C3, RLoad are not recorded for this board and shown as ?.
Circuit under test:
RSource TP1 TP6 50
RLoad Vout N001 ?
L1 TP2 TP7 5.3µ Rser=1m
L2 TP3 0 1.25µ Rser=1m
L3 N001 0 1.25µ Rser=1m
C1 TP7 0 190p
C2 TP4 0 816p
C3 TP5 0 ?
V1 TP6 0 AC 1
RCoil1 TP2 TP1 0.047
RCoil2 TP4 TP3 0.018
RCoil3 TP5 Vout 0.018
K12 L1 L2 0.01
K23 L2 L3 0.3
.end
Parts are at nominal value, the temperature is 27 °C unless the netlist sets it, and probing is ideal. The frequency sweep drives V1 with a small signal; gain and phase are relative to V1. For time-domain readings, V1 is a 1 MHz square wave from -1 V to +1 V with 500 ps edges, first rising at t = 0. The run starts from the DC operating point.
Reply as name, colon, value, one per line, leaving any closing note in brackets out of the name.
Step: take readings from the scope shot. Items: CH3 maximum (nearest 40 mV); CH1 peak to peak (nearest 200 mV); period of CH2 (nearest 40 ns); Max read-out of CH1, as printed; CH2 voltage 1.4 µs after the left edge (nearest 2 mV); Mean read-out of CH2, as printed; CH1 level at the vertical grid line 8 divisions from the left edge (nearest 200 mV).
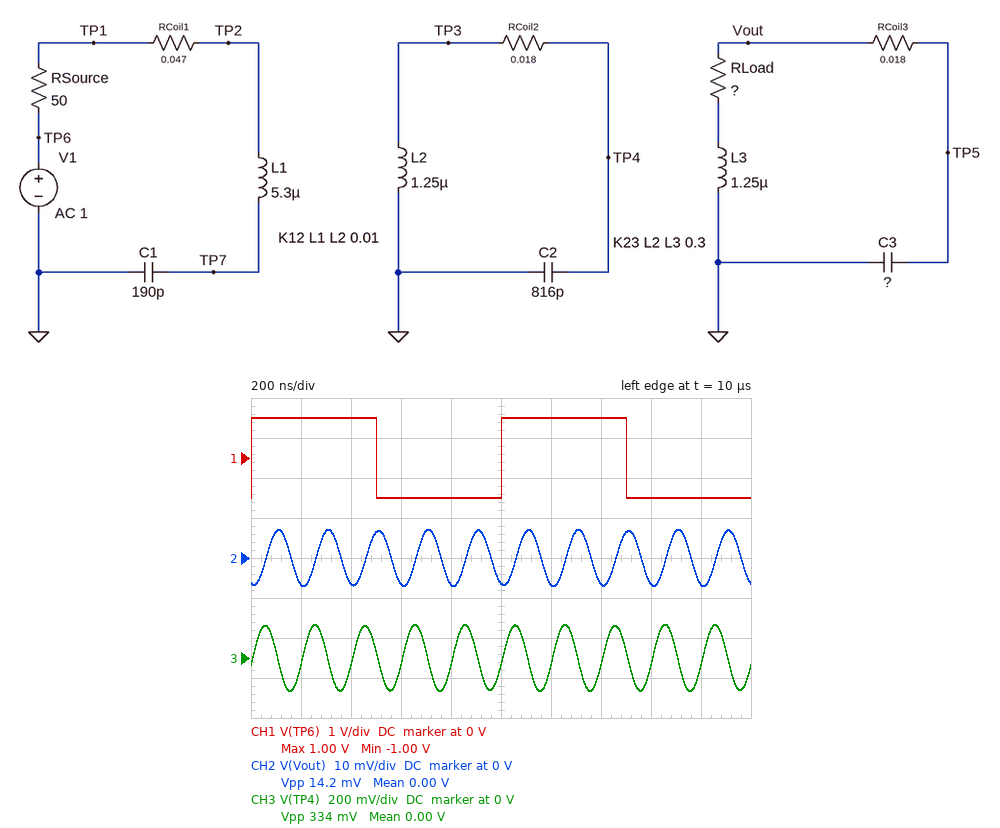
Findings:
CH3 maximum: 160 mV
CH1 peak to peak: 2.0 V
period of CH2: 200 ns
Max read-out of CH1, as printed: 1.00 V
CH2 voltage 1.4 µs after the left edge: -6 mV
Mean read-out of CH2, as printed: 0.00 V
CH1 level at the vertical grid line 8 divisions from the left edge: -1.0 V
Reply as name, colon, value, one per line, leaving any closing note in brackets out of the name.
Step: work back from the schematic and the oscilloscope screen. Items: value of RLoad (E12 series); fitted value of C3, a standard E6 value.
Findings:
value of RLoad: 150 Ω
fitted value of C3, a standard E6 value: 1.5 nF
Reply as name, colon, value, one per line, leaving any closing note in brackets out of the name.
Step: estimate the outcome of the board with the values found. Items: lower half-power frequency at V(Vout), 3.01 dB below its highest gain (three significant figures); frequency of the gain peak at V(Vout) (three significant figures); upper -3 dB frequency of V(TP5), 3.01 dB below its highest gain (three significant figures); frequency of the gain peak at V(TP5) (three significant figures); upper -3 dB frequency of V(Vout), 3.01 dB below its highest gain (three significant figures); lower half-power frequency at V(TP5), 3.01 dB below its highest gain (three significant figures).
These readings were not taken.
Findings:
lower half-power frequency at V(Vout), 3.01 dB below its highest gain: 4.93 MHz
frequency of the gain peak at V(Vout): 4.99 MHz
upper -3 dB frequency of V(TP5), 3.01 dB below its highest gain: 5.05 MHz
frequency of the gain peak at V(TP5): 4.99 MHz
upper -3 dB frequency of V(Vout), 3.01 dB below its highest gain: 5.05 MHz
lower half-power frequency at V(TP5), 3.01 dB below its highest gain: 4.93 MHz
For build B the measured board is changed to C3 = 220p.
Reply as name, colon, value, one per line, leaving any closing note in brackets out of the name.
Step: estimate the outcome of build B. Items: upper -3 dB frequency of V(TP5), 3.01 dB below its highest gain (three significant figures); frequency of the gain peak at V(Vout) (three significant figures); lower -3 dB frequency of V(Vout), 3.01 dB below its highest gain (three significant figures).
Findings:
upper -3 dB frequency of V(TP5), 3.01 dB below its highest gain: 5.00 MHz
frequency of the gain peak at V(Vout): 4.96 MHz
lower -3 dB frequency of V(Vout), 3.01 dB below its highest gain: 4.92 MHz
